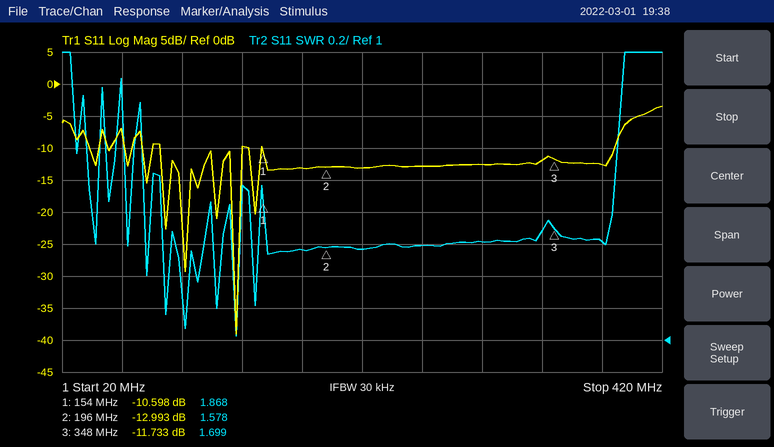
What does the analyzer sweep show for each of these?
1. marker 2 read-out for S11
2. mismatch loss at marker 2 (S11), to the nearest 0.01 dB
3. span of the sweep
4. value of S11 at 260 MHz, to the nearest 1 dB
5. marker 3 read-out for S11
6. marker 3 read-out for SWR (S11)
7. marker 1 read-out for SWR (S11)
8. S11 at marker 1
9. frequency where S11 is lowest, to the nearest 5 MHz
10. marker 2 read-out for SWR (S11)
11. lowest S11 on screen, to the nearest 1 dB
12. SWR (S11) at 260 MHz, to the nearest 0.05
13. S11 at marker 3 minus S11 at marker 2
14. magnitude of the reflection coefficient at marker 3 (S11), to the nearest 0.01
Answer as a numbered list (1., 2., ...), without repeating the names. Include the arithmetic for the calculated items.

1. -12.993 dB
2. −10 log10(1 − 10^(-12.993/10)) ≈ 0.22 dB
3. 400 MHz
4. -13 dB
5. -11.733 dB
6. 1.699
7. 1.868
8. -10.598 dB
9. 135 MHz
10. 1.578
11. -39 dB
12. 1.60
13. -11.733 − (-12.993) = 1.260 dB
14. 10^(-11.733/20) ≈ 0.26
